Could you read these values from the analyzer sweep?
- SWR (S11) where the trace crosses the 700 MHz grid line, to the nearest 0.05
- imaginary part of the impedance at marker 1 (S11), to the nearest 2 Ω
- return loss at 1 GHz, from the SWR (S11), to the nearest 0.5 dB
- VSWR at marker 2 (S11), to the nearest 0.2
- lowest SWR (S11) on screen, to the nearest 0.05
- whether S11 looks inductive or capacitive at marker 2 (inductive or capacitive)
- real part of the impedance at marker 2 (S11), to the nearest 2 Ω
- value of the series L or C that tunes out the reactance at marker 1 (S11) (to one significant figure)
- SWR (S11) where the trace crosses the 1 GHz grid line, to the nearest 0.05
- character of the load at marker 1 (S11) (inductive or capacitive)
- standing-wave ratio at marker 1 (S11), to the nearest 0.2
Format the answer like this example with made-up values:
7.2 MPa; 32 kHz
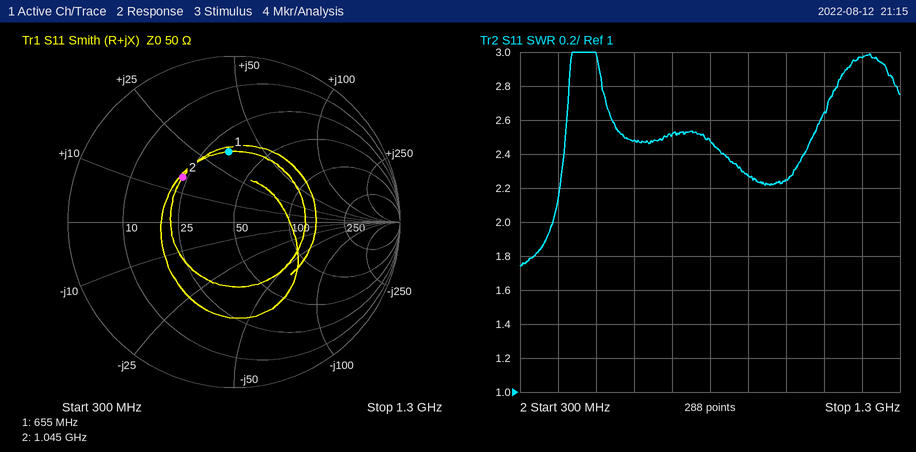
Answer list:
2.50; +34 Ω; 8.5 dB; 2.4; 1.75; inductive; 24 Ω; 7 pF; 2.25; inductive; 2.4
